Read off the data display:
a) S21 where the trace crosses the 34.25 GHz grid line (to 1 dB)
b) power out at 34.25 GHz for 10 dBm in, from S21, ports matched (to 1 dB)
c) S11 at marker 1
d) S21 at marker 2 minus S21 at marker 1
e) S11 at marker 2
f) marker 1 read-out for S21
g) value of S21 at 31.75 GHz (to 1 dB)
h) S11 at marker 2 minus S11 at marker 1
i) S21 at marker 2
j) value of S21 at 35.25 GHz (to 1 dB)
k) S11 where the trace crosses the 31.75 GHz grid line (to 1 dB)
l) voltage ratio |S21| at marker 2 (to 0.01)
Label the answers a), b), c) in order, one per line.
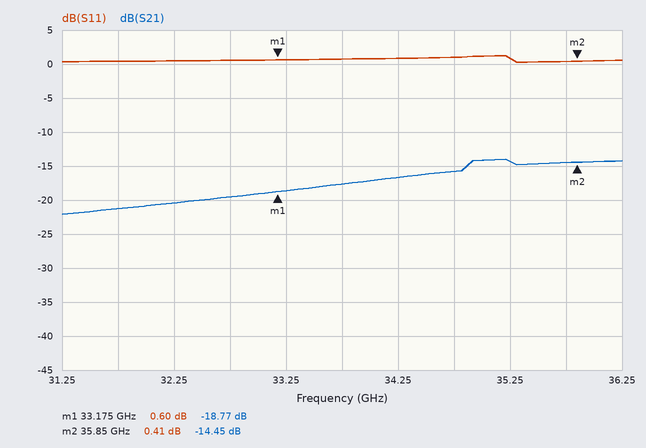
a) -17 dB
b) -7 dBm
c) 0.60 dB
d) 4.32 dB
e) 0.41 dB
f) -18.77 dB
g) -21 dB
h) -0.19 dB
i) -14.45 dB
j) -14 dB
k) 0 dB
l) 0.19
